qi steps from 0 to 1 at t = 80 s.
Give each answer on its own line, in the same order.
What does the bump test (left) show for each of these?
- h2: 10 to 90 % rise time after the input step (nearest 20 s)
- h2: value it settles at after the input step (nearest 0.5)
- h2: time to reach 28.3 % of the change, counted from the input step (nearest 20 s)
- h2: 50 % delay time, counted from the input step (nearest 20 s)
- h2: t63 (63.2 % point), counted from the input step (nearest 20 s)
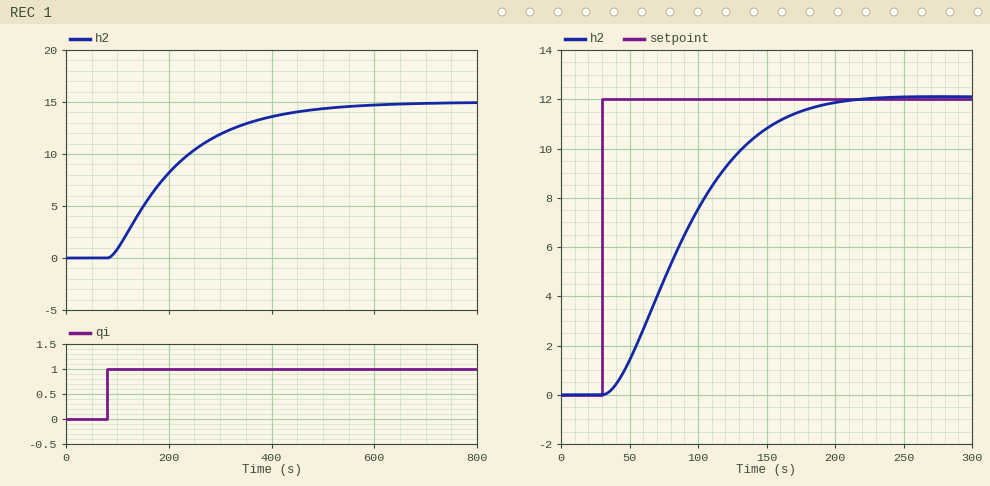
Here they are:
280 s
15.0
60 s
100 s
140 s
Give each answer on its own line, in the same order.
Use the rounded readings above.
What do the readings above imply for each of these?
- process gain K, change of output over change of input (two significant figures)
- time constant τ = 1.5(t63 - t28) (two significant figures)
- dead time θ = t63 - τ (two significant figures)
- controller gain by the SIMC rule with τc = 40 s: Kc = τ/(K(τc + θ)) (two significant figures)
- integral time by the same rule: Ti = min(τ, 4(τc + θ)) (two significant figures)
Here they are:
15
120 s
20 s
0.13
120 s
